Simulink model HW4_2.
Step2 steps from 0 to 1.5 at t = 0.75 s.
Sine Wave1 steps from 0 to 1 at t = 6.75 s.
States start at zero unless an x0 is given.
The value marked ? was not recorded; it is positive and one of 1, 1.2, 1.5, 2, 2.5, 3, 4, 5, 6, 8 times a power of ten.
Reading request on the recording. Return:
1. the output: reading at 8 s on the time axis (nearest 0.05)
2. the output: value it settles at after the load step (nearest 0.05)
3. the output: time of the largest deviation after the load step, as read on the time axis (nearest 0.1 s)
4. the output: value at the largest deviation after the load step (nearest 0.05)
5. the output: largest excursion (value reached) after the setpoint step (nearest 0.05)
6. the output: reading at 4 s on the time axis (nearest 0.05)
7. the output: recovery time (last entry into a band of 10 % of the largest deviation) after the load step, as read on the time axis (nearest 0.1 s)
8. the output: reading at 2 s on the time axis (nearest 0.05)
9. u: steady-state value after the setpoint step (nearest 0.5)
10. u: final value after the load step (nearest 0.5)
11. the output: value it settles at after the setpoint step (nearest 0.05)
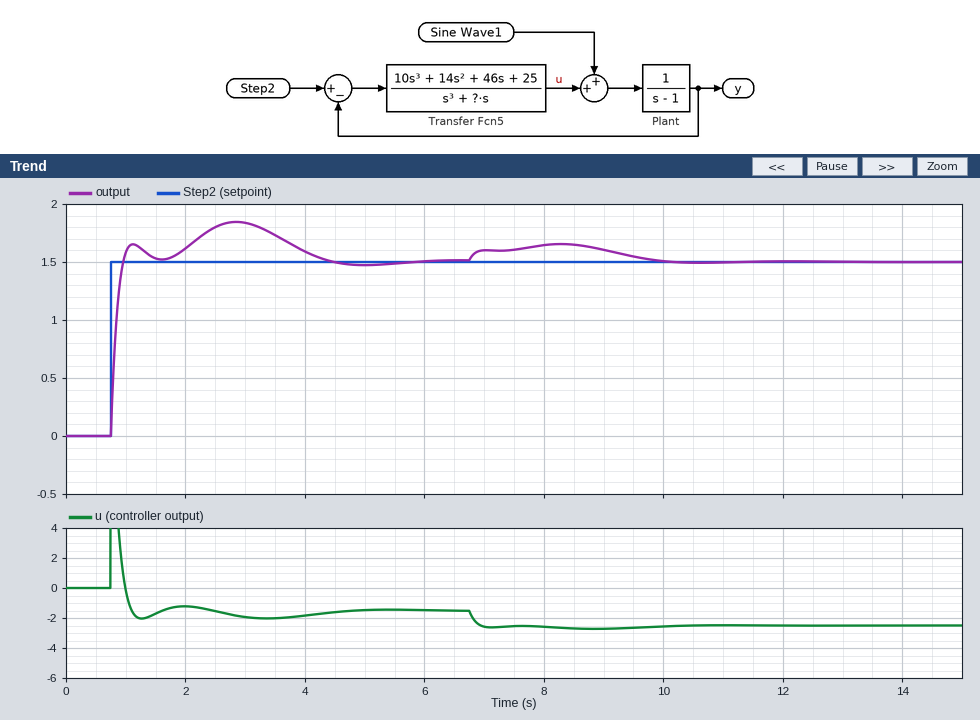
1.65
1.50
8.3 s
1.65
1.85
1.60
9.9 s
1.60
-1.5
-2.5
1.50
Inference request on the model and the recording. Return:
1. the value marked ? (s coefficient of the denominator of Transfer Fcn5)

8
